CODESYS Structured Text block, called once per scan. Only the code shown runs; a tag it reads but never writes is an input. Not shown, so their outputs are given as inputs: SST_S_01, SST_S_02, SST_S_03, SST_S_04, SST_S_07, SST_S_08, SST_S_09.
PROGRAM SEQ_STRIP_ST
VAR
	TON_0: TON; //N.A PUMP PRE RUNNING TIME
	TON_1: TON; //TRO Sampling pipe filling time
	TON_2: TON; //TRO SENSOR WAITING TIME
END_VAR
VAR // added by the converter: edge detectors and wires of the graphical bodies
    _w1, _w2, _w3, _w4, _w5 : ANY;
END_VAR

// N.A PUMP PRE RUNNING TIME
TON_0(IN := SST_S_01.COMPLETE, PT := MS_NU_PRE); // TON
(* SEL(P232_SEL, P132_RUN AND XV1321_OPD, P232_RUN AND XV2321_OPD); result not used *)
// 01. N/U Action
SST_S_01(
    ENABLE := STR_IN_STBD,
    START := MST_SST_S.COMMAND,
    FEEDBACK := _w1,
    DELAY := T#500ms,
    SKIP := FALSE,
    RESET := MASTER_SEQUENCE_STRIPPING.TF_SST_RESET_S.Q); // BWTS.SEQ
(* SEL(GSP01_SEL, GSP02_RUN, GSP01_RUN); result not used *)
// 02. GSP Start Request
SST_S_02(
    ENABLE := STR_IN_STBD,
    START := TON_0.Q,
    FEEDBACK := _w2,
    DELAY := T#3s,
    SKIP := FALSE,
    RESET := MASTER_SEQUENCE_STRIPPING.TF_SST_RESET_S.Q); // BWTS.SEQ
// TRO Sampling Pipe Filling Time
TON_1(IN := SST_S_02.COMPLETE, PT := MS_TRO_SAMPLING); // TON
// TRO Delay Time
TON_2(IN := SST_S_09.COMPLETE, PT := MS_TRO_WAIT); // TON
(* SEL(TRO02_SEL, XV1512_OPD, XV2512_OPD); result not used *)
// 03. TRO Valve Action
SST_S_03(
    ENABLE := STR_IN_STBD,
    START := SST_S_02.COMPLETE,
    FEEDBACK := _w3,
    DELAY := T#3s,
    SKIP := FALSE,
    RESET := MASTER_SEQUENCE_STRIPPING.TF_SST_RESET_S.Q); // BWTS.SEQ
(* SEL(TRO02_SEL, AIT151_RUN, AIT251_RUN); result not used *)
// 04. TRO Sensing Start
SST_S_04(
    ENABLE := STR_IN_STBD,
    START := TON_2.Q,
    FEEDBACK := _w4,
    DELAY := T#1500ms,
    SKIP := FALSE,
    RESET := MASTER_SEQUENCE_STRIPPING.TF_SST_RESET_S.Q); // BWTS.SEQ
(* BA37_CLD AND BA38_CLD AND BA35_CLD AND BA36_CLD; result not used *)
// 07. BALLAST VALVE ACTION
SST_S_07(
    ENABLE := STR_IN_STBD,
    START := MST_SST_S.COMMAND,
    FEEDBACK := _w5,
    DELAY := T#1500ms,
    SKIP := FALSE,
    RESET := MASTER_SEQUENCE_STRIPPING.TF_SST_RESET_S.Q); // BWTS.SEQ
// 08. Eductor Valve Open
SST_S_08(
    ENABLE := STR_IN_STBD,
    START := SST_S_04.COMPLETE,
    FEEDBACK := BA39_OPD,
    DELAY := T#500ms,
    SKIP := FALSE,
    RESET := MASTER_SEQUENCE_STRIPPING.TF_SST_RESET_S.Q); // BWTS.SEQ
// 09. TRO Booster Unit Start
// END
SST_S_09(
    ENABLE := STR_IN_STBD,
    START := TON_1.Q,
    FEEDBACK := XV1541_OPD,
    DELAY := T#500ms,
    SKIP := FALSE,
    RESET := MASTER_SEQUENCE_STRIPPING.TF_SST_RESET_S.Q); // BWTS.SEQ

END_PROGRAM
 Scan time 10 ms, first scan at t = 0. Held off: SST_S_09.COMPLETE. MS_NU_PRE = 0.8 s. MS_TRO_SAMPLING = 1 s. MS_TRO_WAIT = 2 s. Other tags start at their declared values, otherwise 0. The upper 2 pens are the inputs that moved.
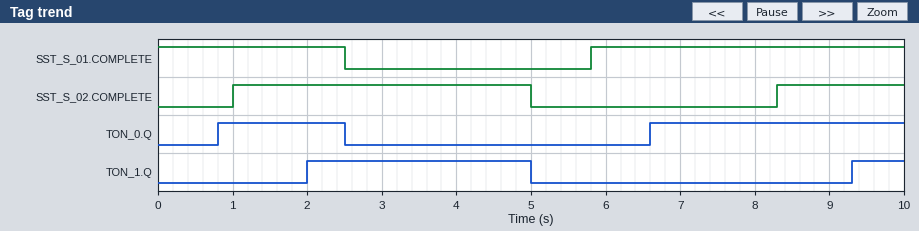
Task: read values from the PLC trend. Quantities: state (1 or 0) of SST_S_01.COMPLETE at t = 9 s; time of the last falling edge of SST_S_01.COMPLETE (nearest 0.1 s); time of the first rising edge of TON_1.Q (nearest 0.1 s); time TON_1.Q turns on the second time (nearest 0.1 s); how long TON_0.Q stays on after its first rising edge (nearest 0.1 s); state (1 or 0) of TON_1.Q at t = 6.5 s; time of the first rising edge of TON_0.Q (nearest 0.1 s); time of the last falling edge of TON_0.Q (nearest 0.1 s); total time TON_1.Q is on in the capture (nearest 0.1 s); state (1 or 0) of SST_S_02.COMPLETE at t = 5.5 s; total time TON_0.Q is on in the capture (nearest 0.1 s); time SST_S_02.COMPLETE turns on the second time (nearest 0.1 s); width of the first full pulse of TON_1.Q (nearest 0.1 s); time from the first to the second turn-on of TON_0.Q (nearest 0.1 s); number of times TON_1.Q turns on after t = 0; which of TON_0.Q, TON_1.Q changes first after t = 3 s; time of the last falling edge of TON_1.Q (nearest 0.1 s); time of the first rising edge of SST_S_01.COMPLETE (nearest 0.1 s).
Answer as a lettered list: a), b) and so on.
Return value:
a) 1
b) 2.5 s
c) 2.0 s
d) 9.3 s
e) 1.7 s
f) 0
g) 0.8 s
h) 2.5 s
i) 3.7 s
j) 0
k) 5.1 s
l) 8.3 s
m) 3.0 s
n) 5.8 s
o) 2
p) TON_1.Q
q) 5.0 s
r) 5.8 s
